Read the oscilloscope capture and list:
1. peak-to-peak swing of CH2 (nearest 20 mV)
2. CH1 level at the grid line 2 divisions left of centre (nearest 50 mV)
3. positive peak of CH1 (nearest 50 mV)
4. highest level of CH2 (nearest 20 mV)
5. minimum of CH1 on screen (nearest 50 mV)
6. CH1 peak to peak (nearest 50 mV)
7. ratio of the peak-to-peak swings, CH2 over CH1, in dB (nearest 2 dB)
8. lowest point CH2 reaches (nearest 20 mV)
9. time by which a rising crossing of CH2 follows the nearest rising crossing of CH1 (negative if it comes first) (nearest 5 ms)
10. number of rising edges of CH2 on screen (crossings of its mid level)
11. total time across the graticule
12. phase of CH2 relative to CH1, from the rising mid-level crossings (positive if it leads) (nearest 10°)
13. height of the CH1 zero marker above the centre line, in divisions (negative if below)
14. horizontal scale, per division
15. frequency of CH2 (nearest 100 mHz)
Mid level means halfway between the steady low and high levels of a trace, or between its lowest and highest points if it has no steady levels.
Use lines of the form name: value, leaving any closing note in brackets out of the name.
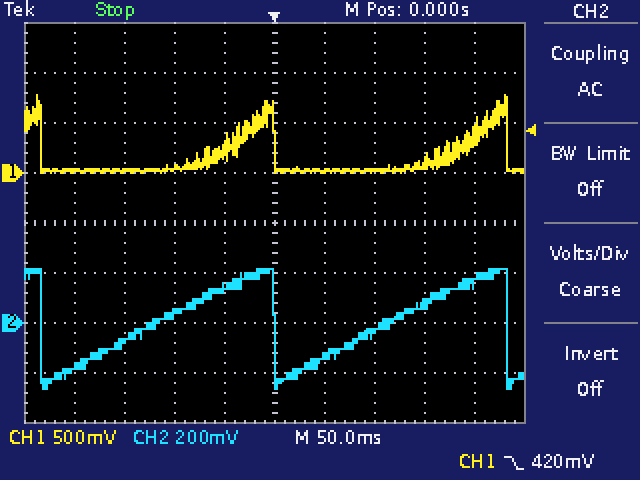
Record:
peak-to-peak swing of CH2: 480 mV
CH1 level at the grid line 2 divisions left of centre: 50 mV
positive peak of CH1: 800 mV
highest level of CH2: 220 mV
minimum of CH1 on screen: 0 mV
CH1 peak to peak: 800 mV
ratio of the peak-to-peak swings, CH2 over CH1, in dB: -4 dB
lowest point CH2 reaches: -260 mV
time by which a rising crossing of CH2 follows the nearest rising crossing of CH1 (negative if it comes first): -100 ms
number of rising edges of CH2 on screen: 2
total time across the graticule: 500 ms
phase of CH2 relative to CH1, from the rising mid-level crossings (positive if it leads): +150°
height of the CH1 zero marker above the centre line, in divisions: +1.0 div
horizontal scale, per division: 50 ms
frequency of CH2: 4.3 Hz
